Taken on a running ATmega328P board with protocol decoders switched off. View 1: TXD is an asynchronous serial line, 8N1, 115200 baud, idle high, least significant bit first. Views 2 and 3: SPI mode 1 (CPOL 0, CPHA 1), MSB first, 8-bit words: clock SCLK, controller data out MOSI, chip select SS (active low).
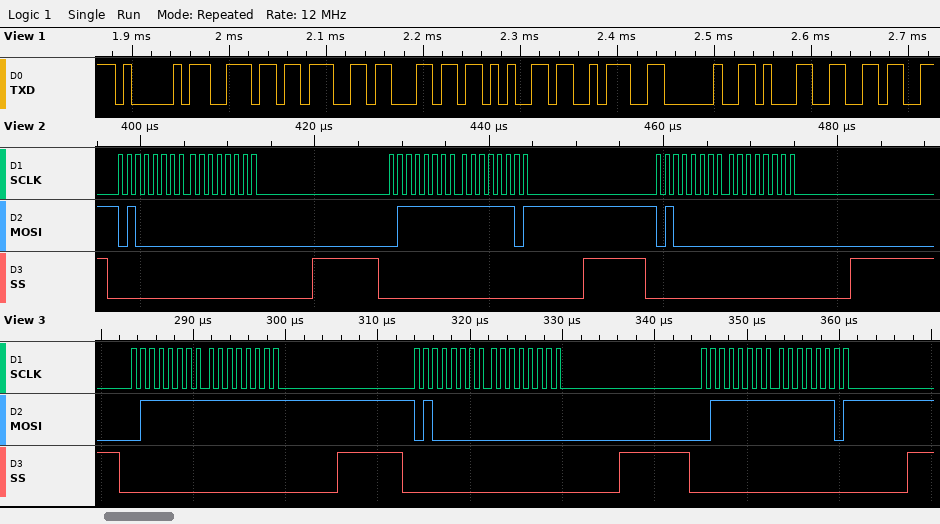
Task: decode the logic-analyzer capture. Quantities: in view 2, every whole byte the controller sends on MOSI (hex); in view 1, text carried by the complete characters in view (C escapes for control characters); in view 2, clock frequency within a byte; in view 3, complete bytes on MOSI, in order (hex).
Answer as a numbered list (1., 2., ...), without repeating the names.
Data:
1. 40 00 7F FD 40 00
2. "Angle: 16"
3. 1 MHz
4. 7F FF 40 00 7F FD
